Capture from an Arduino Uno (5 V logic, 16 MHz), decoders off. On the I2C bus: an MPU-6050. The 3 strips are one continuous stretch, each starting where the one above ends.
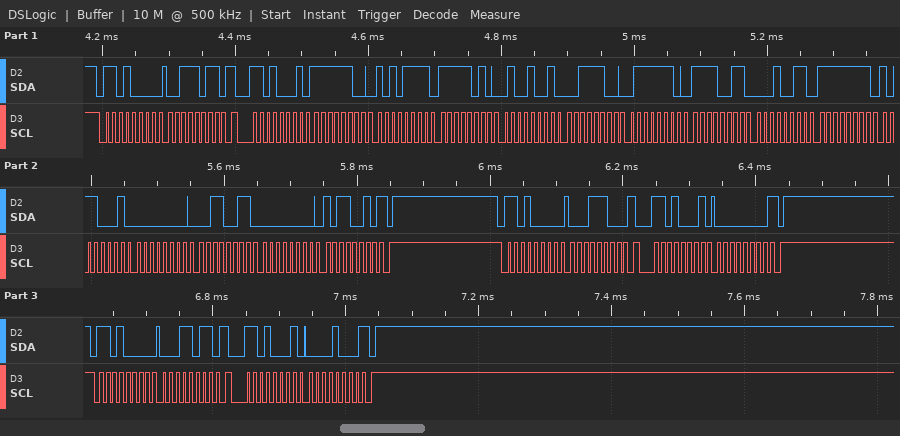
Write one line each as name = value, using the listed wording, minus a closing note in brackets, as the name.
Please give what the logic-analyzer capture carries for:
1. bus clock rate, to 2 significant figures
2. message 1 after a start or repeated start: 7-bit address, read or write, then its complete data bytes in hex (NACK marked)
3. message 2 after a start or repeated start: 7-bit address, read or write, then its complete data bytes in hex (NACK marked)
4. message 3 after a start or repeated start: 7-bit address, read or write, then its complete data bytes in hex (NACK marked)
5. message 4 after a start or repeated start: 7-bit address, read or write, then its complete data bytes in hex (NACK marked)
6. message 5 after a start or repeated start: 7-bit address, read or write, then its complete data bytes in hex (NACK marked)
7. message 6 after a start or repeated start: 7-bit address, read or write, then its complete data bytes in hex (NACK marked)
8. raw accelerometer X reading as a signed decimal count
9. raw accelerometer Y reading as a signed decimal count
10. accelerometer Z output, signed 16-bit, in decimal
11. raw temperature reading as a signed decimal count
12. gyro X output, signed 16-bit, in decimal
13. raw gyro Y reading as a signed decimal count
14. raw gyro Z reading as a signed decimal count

bus clock rate, to 2 significant figures = 100 kHz
message 1 after a start or repeated start: 7-bit address, read or write, then its complete data bytes in hex = 0x68 write: 3B
message 2 after a start or repeated start: 7-bit address, read or write, then its complete data bytes in hex = 0x68 read: FC AF FA 49 3C 7E F3 13 FF B1 00 33 00 B2 NACK
message 3 after a start or repeated start: 7-bit address, read or write, then its complete data bytes in hex = 0x68 write: 1C
message 4 after a start or repeated start: 7-bit address, read or write, then its complete data bytes in hex = 0x68 read: 00 NACK
message 5 after a start or repeated start: 7-bit address, read or write, then its complete data bytes in hex = 0x68 write: 1B
message 6 after a start or repeated start: 7-bit address, read or write, then its complete data bytes in hex = 0x68 read: 08 NACK
raw accelerometer X reading as a signed decimal count = -849
raw accelerometer Y reading as a signed decimal count = -1463
accelerometer Z output, signed 16-bit, in decimal = 15486
raw temperature reading as a signed decimal count = -3309
gyro X output, signed 16-bit, in decimal = -79
raw gyro Y reading as a signed decimal count = 51
raw gyro Z reading as a signed decimal count = 178
